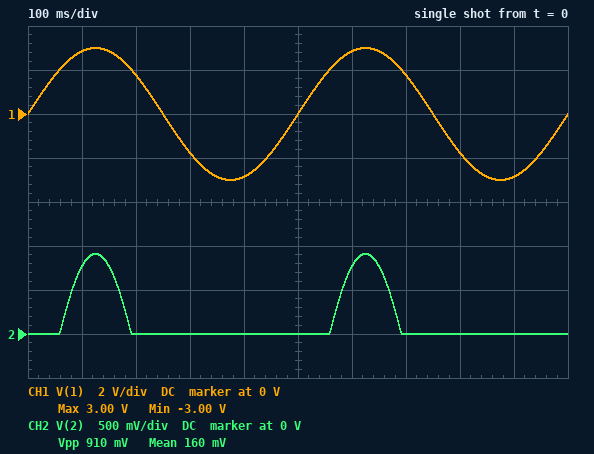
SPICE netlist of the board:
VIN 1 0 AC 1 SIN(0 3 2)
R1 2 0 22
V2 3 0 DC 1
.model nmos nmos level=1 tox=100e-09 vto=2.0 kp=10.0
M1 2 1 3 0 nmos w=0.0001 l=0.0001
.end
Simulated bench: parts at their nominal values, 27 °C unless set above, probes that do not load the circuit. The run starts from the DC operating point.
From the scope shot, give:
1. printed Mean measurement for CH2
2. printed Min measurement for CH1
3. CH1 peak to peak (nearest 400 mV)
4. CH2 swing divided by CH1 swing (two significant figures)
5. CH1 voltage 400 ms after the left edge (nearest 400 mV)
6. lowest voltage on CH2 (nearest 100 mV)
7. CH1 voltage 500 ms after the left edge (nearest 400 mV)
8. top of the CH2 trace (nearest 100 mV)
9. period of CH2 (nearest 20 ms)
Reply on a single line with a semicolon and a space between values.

160 mV; -3.00 V; 6.0 V; 0.15; -2.8 V; 0 V; 0 V; 900 mV; 500 ms
